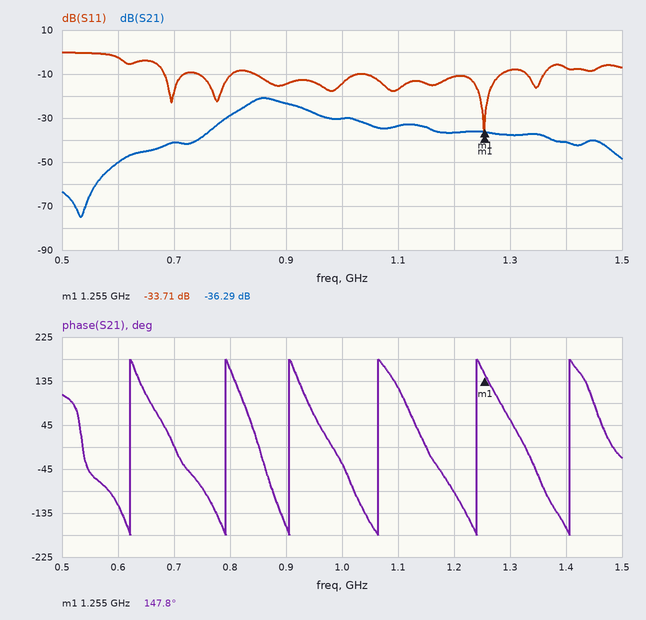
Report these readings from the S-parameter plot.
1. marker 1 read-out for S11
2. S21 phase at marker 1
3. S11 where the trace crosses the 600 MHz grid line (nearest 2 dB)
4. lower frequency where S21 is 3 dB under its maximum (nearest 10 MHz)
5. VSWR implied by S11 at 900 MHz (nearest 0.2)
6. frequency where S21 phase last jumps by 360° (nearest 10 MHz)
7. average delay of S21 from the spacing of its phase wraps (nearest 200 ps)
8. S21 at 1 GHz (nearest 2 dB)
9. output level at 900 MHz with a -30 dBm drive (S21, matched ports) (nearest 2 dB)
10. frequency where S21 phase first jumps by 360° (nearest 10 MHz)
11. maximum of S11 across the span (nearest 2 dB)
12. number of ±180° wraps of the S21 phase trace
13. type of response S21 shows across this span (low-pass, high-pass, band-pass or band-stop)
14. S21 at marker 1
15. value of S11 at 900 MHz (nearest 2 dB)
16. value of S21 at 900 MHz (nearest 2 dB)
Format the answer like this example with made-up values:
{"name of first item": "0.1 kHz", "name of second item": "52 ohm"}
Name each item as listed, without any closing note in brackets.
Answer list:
{"marker 1 read-out for S11": "-33.71 dB", "S21 phase at marker 1": "147.8°", "S11 where the trace crosses the 600 MHz grid line": "-2 dB", "lower frequency where S21 is 3 dB under its maximum": "830 MHz", "VSWR implied by S11 at 900 MHz": "1.4", "frequency where S21 phase last jumps by 360°": "1.41 GHz", "average delay of S21 from the spacing of its phase wraps": "6.4 ns", "S21 at 1 GHz": "-30 dB", "output level at 900 MHz with a -30 dBm drive (S21, matched ports)": "-54 dBm", "frequency where S21 phase first jumps by 360°": "620 MHz", "maximum of S11 across the span": "0 dB", "number of ±180° wraps of the S21 phase trace": "6", "type of response S21 shows across this span": "band-pass", "S21 at marker 1": "-36.29 dB", "value of S11 at 900 MHz": "-14 dB", "value of S21 at 900 MHz": "-24 dB"}
